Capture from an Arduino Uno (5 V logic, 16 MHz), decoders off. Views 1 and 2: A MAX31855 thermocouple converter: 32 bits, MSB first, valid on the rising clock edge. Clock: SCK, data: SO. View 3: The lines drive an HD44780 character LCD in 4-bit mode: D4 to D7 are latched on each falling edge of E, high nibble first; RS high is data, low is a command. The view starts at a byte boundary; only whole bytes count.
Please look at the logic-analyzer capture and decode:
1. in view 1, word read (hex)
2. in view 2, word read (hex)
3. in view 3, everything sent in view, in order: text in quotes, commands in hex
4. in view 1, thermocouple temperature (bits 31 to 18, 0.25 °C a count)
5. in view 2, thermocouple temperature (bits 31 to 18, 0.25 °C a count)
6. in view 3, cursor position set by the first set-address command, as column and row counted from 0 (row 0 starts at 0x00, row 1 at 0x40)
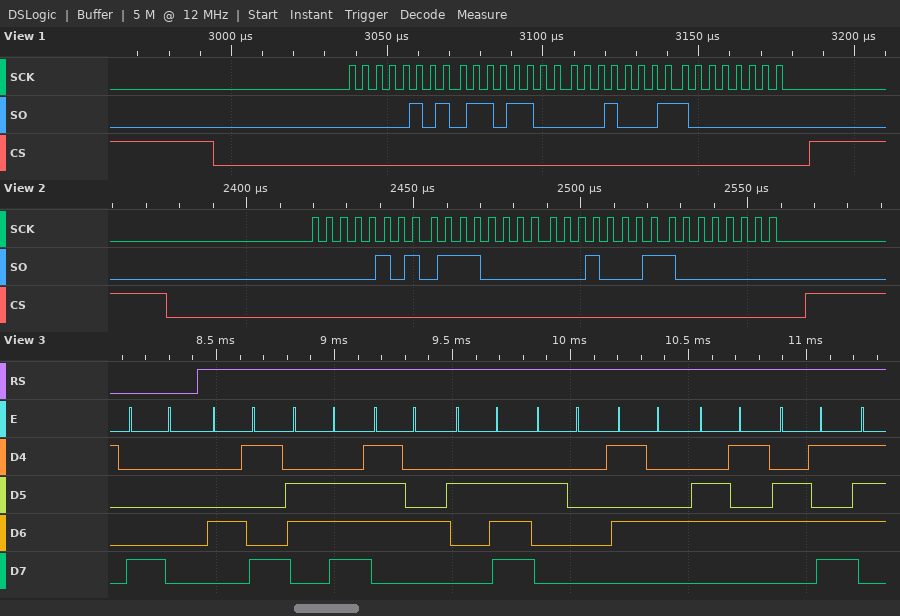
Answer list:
0x056C1180
0x05701180
0x80 "Int. Tem"
86.75 °C
87.00 °C
column 0, row 0
